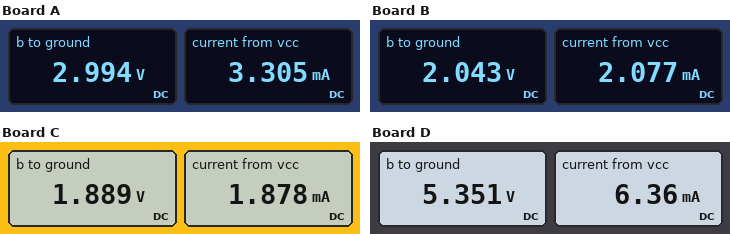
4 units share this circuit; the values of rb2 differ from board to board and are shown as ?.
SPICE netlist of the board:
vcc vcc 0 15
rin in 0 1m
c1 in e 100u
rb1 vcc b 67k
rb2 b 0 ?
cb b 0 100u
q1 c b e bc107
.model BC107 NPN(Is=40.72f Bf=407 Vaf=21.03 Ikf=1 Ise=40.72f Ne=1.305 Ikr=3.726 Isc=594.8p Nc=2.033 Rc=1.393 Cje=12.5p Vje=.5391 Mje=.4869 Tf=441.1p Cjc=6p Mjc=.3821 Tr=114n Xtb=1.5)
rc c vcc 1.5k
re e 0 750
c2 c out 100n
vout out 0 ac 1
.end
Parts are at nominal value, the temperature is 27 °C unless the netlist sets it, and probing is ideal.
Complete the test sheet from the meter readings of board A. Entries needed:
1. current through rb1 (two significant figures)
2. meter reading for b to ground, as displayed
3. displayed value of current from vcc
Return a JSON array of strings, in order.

["180 µA", "2.994 V", "3.305 mA"]
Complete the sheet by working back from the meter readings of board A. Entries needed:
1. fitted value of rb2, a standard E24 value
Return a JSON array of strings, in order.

["18 kΩ"]
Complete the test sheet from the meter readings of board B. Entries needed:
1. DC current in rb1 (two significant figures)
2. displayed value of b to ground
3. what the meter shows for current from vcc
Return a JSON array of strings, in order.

["190 µA", "2.043 V", "2.077 mA"]
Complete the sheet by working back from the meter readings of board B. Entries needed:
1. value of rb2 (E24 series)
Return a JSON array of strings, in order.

["11 kΩ"]
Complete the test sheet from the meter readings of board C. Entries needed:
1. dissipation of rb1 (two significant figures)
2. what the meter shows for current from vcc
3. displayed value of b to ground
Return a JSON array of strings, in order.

["2.6 mW", "1.878 mA", "1.889 V"]
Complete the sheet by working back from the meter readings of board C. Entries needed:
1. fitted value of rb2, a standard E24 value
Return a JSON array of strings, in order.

["10 kΩ"]
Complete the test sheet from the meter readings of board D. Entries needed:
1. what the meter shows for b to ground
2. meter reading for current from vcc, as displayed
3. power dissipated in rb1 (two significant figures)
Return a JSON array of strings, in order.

["5.351 V", "6.36 mA", "1.4 mW"]
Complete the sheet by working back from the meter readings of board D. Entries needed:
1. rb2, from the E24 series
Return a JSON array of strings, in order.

["47 kΩ"]
